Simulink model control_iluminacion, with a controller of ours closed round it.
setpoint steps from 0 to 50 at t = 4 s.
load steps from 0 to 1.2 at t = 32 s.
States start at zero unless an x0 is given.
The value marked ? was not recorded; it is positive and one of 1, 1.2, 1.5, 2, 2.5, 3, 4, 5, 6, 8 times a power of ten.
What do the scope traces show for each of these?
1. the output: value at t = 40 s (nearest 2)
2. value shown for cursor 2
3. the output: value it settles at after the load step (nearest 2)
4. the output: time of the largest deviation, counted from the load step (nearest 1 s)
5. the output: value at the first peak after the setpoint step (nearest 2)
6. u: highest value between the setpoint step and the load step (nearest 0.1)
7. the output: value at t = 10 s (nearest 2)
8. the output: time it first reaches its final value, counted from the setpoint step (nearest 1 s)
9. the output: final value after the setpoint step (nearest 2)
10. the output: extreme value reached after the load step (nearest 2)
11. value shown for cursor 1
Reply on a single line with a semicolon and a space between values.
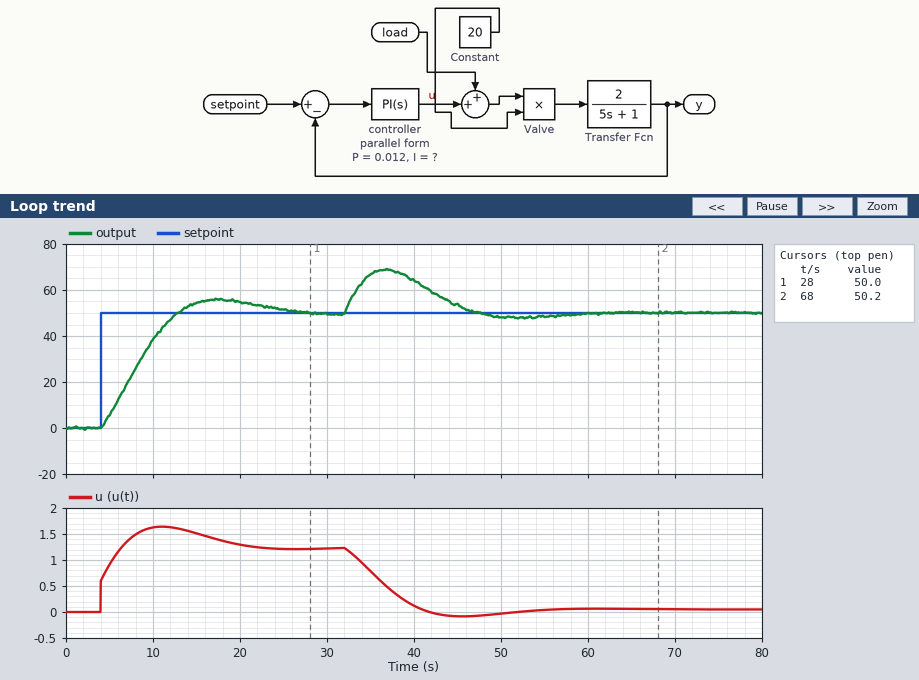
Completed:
64; 50.2; 50; 5 s; 56; 1.6; 38; 9 s; 50; 68; 50.0
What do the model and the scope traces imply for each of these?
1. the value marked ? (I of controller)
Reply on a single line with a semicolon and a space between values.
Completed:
0.008
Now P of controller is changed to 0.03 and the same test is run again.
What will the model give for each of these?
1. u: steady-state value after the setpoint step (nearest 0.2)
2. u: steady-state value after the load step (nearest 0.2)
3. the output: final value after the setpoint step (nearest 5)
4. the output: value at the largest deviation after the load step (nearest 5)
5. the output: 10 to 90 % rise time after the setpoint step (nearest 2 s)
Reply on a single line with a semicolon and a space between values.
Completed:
1.2; 0.0; 50; 65; 6 s
